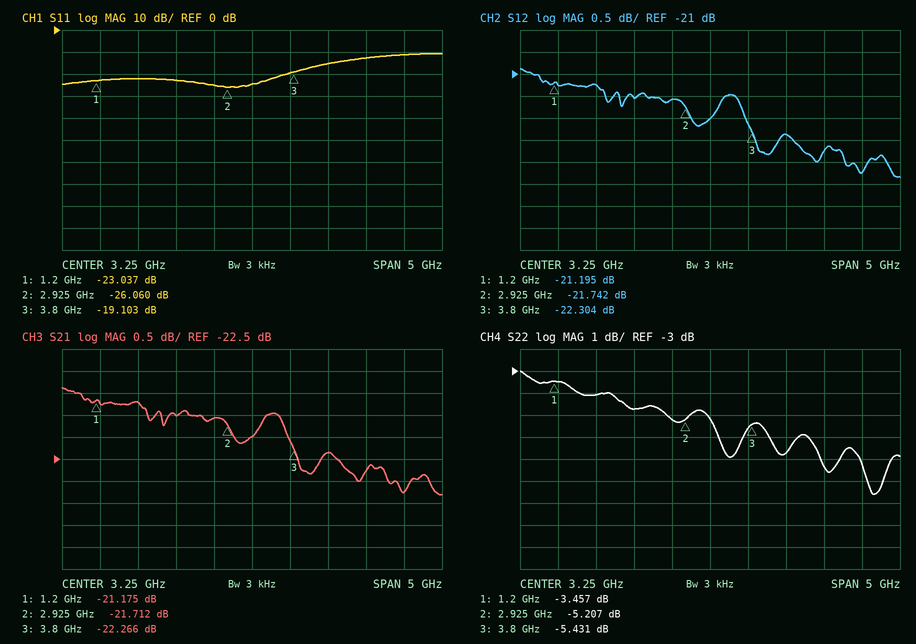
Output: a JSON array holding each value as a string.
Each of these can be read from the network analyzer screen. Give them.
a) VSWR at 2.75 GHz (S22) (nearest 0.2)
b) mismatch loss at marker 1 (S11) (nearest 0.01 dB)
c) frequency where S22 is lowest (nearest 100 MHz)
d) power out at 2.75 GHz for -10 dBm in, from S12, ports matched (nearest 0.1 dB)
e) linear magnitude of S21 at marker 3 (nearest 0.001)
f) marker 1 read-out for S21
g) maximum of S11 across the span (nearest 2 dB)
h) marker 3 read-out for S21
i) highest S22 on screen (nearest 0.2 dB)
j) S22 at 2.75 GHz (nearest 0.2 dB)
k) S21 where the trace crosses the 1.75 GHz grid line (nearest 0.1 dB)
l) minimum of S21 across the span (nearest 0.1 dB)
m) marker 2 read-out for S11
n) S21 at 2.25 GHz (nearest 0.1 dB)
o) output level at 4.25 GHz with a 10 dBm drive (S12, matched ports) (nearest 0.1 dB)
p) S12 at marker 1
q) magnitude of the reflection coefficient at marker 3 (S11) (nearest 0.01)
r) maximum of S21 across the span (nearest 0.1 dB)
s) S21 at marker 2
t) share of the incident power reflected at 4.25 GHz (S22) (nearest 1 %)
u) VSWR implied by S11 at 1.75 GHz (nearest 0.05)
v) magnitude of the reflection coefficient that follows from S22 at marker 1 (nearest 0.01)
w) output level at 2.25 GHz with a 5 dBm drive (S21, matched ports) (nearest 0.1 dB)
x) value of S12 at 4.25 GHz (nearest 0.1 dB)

["3.4", "0.02 dB", "5.4 GHz", "-31.6 dBm", "0.077", "-21.175 dB", "-10 dB", "-22.266 dB", "-3.0 dB", "-5.2 dB", "-21.2 dB", "-23.3 dB", "-26.060 dB", "-21.5 dB", "-12.4 dBm", "-21.195 dB", "0.11", "-20.9 dB", "-21.712 dB", "21 %", "1.15", "0.67", "-16.5 dBm", "-22.4 dB"]
